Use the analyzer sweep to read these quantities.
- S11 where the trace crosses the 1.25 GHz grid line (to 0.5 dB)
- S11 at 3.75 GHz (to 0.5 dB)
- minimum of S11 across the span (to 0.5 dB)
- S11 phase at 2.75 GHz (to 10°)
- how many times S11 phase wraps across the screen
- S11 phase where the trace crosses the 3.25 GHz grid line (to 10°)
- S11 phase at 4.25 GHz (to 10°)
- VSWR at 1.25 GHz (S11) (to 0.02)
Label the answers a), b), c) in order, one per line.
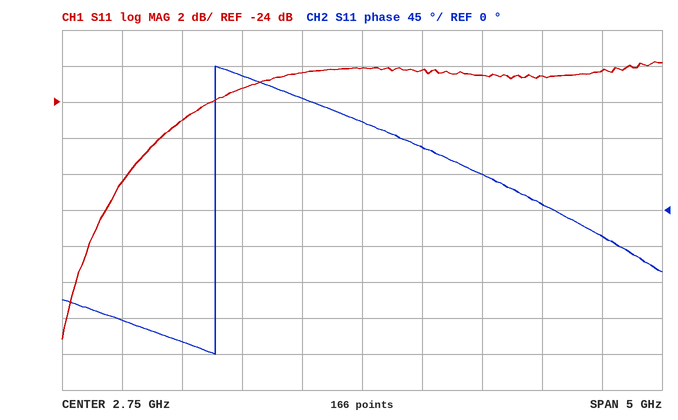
a) -25.0 dB
b) -22.5 dB
c) -37.0 dB
d) 110°
e) 1
f) 80°
g) 10°
h) 1.12
